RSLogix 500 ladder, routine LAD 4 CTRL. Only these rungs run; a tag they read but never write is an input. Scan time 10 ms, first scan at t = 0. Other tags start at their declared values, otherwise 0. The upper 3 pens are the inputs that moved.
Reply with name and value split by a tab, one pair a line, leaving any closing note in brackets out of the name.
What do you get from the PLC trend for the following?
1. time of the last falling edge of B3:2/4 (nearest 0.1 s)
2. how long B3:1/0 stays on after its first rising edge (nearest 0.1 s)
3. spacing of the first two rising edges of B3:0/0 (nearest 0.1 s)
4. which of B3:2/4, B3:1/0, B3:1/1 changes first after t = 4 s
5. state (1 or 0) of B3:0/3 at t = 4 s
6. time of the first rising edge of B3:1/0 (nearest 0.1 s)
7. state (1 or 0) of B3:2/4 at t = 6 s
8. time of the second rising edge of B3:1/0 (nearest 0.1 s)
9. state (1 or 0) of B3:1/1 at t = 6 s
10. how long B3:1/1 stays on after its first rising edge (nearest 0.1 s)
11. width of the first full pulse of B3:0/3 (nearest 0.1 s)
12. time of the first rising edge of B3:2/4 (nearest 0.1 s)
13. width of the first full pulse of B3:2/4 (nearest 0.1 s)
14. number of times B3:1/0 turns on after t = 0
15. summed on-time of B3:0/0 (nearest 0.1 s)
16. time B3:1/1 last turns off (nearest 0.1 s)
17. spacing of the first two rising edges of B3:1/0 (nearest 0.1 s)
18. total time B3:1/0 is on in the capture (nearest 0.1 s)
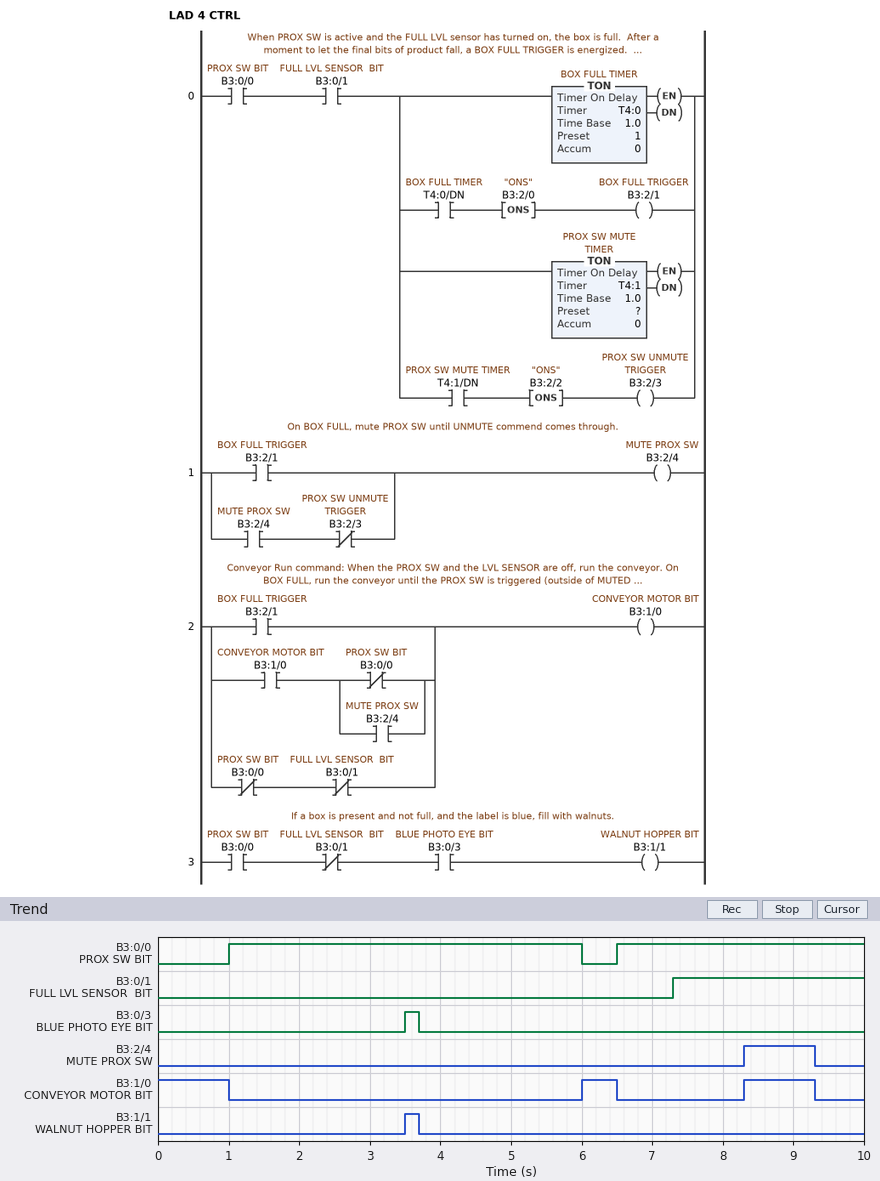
time of the last falling edge of B3:2/4	9.3 s
how long B3:1/0 stays on after its first rising edge	0.5 s
spacing of the first two rising edges of B3:0/0	5.5 s
which of B3:2/4, B3:1/0, B3:1/1 changes first after t = 4 s	B3:1/0
state (1 or 0) of B3:0/3 at t = 4 s	0
time of the first rising edge of B3:1/0	6.0 s
state (1 or 0) of B3:2/4 at t = 6 s	0
time of the second rising edge of B3:1/0	8.3 s
state (1 or 0) of B3:1/1 at t = 6 s	0
how long B3:1/1 stays on after its first rising edge	0.2 s
width of the first full pulse of B3:0/3	0.2 s
time of the first rising edge of B3:2/4	8.3 s
width of the first full pulse of B3:2/4	1.0 s
number of times B3:1/0 turns on after t = 0	2
summed on-time of B3:0/0	8.5 s
time B3:1/1 last turns off	3.7 s
spacing of the first two rising edges of B3:1/0	2.3 s
total time B3:1/0 is on in the capture	2.5 s
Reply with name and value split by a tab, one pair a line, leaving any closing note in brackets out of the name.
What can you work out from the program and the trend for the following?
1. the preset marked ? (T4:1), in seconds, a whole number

the preset marked ? (T4:1), in seconds, a whole number	2 s
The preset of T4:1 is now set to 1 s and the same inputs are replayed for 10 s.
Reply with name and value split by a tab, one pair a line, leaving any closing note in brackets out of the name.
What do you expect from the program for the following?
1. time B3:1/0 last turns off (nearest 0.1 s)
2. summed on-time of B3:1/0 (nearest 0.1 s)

time B3:1/0 last turns off	6.5 s
summed on-time of B3:1/0	3.2 s
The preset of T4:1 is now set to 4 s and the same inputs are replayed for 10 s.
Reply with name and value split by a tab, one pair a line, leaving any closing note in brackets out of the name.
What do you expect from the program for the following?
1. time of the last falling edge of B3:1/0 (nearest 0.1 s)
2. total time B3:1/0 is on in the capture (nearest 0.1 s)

time of the last falling edge of B3:1/0	6.5 s
total time B3:1/0 is on in the capture	3.2 s
